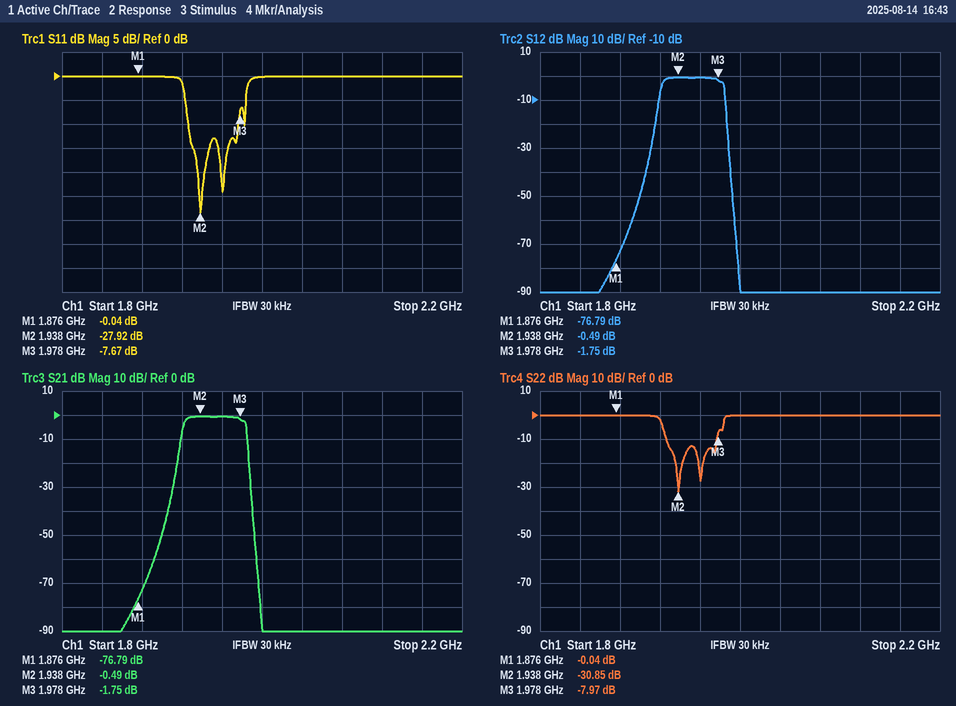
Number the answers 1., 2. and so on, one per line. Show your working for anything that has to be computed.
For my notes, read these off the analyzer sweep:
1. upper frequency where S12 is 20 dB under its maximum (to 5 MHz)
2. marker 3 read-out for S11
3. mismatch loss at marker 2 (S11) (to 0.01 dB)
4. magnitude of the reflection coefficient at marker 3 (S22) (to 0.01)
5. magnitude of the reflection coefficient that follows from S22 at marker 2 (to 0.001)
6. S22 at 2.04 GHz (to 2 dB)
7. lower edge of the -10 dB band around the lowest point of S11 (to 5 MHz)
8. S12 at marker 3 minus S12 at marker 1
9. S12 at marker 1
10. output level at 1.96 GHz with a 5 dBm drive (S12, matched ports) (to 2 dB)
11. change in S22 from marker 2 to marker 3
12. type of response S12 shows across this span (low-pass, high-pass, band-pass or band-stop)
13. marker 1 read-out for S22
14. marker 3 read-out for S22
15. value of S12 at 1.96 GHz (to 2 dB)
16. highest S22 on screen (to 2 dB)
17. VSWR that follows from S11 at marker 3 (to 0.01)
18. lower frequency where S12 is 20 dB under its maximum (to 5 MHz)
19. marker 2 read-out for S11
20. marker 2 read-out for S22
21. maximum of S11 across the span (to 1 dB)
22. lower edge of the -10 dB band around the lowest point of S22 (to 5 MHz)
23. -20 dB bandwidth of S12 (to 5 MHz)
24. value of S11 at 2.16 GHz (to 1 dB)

1. 1.985 GHz
2. -7.67 dB
3. −10 log10(1 − 10^(-27.92/10)) ≈ 0.01 dB
4. 10^(-7.97/20) ≈ 0.40
5. 10^(-30.85/20) ≈ 0.029
6. 0 dB
7. 1.925 GHz
8. -1.75 − (-76.79) = 75.04 dB
9. -76.79 dB
10. 5 dBm + (0 dB) = 4 dBm
11. -7.97 − (-30.85) = 22.88 dB
12. band-pass
13. -0.04 dB
14. -7.97 dB
15. 0 dB
16. 0 dB
17. (1 + 0.4135)/(1 − 0.4135) ≈ 2.41
18. 1.915 GHz
19. -27.92 dB
20. -30.85 dB
21. 0 dB
22. 1.925 GHz
23. 1.985 GHz − 1.915 GHz = 70 MHz
24. 0 dB
